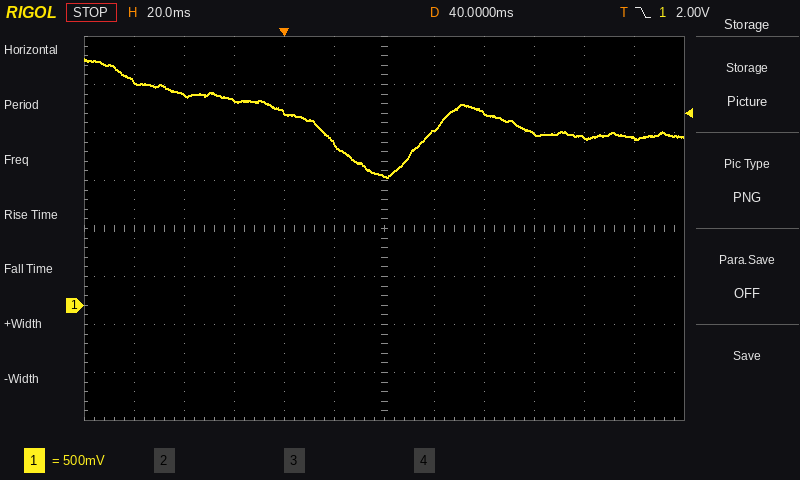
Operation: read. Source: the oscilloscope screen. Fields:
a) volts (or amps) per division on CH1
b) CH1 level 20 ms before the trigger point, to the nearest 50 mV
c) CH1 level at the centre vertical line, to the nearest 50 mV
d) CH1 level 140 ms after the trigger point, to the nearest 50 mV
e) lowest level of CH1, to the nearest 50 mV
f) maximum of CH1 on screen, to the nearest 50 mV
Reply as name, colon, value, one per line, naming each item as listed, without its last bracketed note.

volts (or amps) per division on CH1: 500 mV
CH1 level 20 ms before the trigger point, to the nearest 50 mV: 2.15 V
CH1 level at the centre vertical line, to the nearest 50 mV: 1.35 V
CH1 level 140 ms after the trigger point, to the nearest 50 mV: 1.75 V
lowest level of CH1, to the nearest 50 mV: 1.35 V
maximum of CH1 on screen, to the nearest 50 mV: 2.55 V
